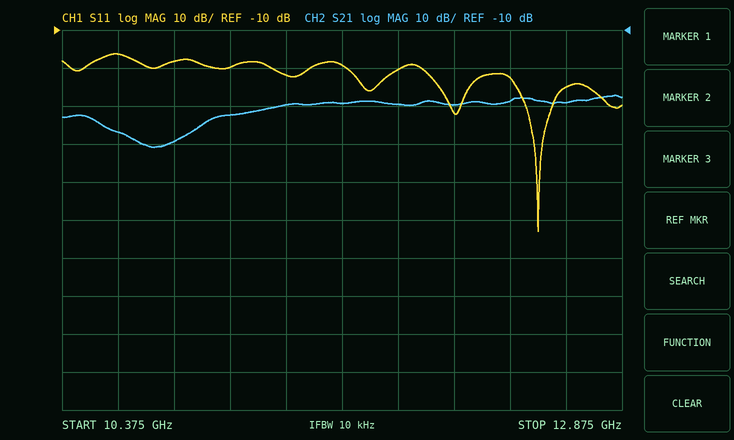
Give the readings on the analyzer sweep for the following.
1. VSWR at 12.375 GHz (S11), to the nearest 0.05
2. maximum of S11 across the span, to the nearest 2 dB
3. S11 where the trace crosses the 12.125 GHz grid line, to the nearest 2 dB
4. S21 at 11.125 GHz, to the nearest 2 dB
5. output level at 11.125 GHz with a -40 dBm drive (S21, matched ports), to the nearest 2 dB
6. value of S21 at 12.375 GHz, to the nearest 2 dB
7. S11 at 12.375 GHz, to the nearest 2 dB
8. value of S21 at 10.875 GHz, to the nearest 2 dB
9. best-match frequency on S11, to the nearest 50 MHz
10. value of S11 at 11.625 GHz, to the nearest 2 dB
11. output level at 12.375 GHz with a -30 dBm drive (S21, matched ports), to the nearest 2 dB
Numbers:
1.15
-16 dB
-32 dB
-32 dB
-72 dBm
-28 dB
-22 dB
-40 dB
12.50 GHz
-20 dB
-58 dBm
